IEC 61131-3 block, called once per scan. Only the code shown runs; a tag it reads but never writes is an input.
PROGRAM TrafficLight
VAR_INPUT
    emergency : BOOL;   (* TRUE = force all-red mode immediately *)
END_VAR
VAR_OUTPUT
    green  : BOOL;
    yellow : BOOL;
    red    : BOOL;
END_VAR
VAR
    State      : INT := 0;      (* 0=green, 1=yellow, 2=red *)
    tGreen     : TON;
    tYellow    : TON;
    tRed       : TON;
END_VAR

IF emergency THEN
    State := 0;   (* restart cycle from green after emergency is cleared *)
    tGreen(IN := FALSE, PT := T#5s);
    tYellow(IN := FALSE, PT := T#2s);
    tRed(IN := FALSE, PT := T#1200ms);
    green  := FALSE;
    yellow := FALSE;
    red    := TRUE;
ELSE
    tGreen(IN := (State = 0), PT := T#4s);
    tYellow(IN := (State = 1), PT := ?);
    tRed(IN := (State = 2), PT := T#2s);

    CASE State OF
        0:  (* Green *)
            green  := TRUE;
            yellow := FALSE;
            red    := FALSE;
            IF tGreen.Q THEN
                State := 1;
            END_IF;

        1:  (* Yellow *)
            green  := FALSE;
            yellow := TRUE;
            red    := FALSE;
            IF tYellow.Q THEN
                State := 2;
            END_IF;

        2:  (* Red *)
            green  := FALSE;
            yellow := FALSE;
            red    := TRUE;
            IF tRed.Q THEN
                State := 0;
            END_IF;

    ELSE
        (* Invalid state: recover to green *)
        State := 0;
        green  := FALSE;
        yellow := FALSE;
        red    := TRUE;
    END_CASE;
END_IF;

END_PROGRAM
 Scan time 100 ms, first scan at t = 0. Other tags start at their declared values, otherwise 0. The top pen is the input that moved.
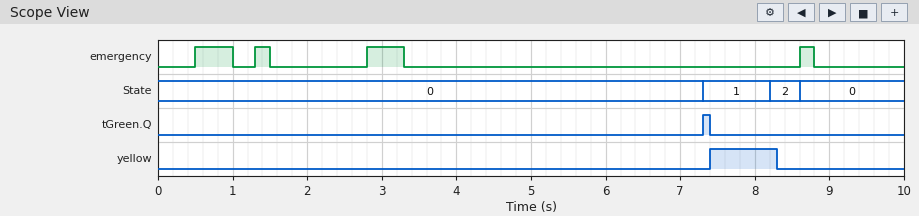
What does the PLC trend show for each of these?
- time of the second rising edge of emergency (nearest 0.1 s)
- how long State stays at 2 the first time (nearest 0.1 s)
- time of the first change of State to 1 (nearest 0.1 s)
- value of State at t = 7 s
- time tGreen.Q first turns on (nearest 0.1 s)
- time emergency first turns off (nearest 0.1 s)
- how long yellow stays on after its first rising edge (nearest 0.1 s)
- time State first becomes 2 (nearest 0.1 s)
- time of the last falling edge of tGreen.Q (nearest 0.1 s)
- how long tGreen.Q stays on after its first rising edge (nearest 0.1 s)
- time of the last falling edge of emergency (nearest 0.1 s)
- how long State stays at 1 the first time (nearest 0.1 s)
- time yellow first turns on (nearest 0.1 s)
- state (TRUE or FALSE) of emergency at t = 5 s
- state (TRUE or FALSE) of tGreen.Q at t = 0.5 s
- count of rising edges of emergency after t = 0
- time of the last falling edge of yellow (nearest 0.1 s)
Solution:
1.3 s
0.4 s
7.3 s
0
7.3 s
1.0 s
0.9 s
8.2 s
7.4 s
0.1 s
8.8 s
0.9 s
7.4 s
FALSE
FALSE
4
8.3 s
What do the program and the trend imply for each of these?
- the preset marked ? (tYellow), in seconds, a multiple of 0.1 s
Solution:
0.8 s
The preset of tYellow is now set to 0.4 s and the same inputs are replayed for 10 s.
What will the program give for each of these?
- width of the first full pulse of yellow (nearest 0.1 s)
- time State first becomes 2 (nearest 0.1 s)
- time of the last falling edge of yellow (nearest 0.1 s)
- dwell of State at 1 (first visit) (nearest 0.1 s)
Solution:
0.5 s
7.8 s
7.9 s
0.5 s
